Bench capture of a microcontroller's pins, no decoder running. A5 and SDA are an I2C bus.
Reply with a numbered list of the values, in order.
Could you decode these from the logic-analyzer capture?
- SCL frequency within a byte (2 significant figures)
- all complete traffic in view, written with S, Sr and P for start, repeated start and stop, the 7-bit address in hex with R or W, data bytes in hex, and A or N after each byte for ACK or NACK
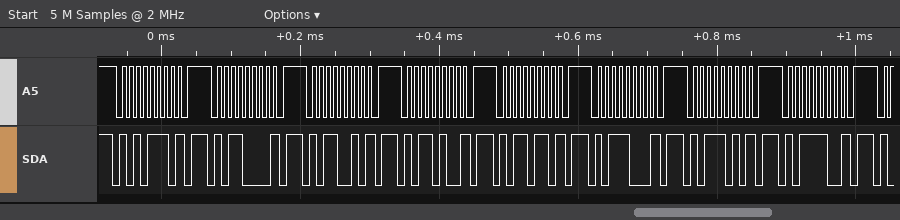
1. 100 kHz
2. S 57W N P S 58W N P S 59W N P S 5AW N P S 5BW N P S 5CW N P S 5DW N P S 5EW N P
